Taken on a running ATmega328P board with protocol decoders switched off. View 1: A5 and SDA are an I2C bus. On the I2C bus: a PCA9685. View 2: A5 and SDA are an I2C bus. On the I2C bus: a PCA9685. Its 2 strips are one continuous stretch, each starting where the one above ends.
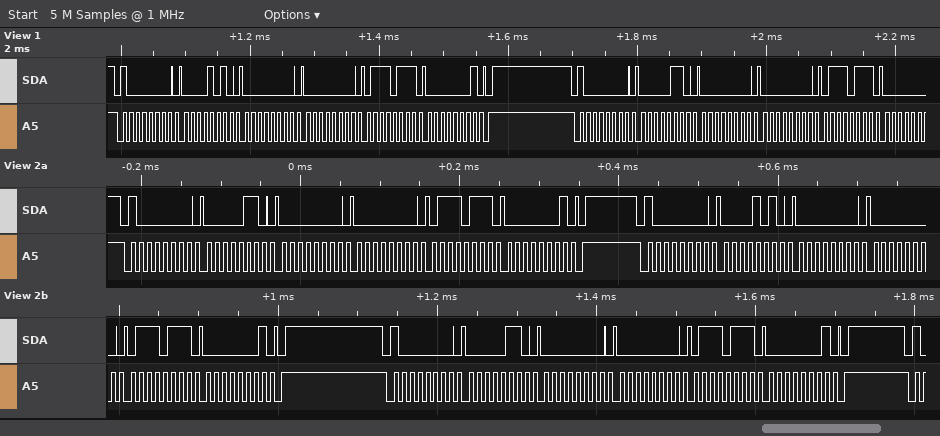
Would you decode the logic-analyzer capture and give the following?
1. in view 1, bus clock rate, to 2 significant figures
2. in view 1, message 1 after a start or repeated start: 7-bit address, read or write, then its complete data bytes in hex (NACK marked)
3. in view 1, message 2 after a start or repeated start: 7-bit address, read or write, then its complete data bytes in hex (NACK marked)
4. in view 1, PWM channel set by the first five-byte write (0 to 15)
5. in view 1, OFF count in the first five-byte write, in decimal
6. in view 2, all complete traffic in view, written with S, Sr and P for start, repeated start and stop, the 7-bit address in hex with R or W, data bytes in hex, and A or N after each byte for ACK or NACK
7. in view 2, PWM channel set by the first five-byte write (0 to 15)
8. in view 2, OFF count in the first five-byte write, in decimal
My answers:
100 kHz
0x40 write: 0A 00 00 77 01
0x40 write: 06 00 00 77
1
375
S 40W A 06 A 00 A 00 A 77 A 01 A P S 40W A 0A A 00 A 00 A 77 A 01 A P S 40W A 06 A 00 A 00 A 77 A 01 A P
0
375
